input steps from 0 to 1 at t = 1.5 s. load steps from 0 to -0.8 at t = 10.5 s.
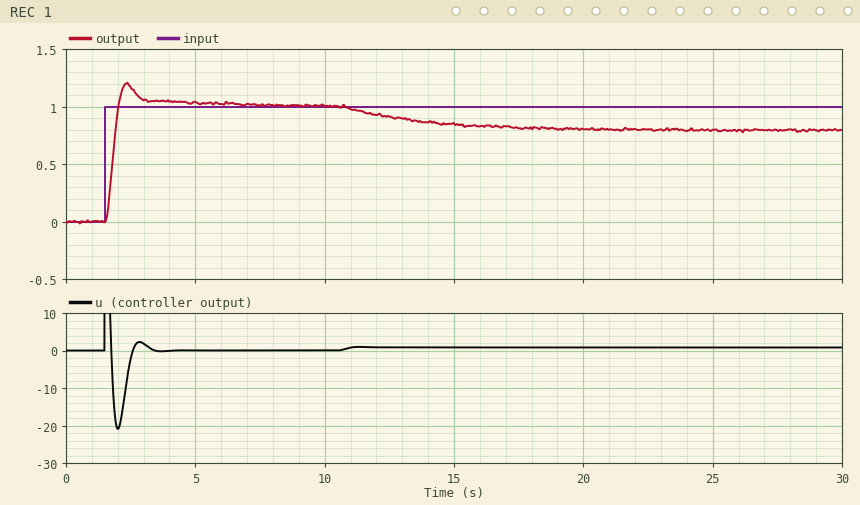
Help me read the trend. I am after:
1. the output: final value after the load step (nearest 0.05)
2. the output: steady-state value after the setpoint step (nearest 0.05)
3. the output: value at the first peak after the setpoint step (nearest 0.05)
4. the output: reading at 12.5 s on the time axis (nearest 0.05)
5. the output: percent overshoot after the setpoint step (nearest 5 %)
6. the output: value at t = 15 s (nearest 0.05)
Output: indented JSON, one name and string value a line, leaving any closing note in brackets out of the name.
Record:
{
  "the output: final value after the load step": "0.80",
  "the output: steady-state value after the setpoint step": "1.00",
  "the output: value at the first peak after the setpoint step": "1.20",
  "the output: reading at 12.5 s on the time axis": "0.90",
  "the output: percent overshoot after the setpoint step": "20 %",
  "the output: value at t = 15 s": "0.85"
}
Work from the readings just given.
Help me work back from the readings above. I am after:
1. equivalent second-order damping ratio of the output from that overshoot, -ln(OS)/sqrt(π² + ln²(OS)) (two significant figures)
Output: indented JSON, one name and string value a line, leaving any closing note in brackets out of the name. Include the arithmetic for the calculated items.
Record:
{
  "equivalent second-order damping ratio of the output from that overshoot, -ln(OS)/sqrt(π² + ln²(OS))": "ln(0.2) = -1.609; 1.609 / sqrt(9.870 + 2.590) = 0.46"
}
